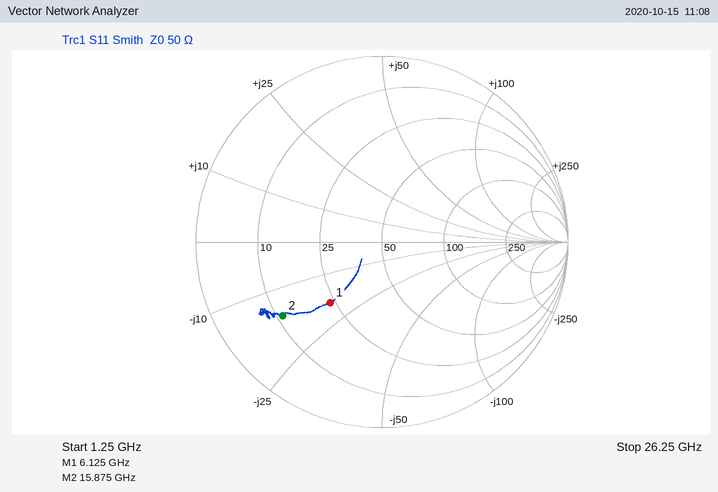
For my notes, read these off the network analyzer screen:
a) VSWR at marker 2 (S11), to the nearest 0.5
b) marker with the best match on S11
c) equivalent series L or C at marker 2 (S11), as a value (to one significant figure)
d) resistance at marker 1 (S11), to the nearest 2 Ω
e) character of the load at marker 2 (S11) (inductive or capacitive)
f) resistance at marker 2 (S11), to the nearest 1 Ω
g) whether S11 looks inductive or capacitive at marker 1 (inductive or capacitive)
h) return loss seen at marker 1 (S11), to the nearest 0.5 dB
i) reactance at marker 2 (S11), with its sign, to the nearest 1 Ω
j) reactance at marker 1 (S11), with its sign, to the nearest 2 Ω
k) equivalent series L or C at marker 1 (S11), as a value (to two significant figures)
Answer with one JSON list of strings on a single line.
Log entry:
["5.0", "marker 1", "600 fF", "24 Ω", "capacitive", "11 Ω", "capacitive", "7.5 dB", "-16 Ω", "-18 Ω", "1.4 pF"]
